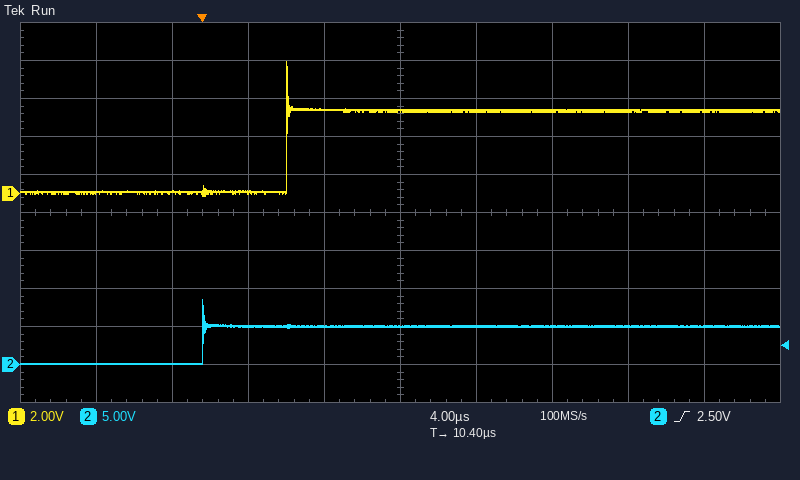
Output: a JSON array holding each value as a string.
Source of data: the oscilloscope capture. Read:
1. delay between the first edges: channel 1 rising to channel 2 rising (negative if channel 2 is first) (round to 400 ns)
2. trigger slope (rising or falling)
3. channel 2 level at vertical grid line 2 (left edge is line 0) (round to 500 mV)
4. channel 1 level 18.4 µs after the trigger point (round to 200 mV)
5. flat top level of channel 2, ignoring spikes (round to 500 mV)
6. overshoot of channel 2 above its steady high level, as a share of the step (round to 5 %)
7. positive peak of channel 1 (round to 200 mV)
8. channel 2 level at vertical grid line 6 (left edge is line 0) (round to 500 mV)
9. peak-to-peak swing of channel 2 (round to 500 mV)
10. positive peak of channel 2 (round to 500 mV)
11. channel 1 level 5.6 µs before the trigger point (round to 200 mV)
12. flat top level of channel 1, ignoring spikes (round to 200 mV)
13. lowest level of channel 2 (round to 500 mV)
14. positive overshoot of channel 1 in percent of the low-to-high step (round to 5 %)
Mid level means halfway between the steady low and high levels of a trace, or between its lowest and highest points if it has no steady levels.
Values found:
["-4.4 µs", "rising", "0.0 V", "4.4 V", "5.0 V", "70 %", "7.0 V", "5.0 V", "8.5 V", "8.5 V", "0.0 V", "4.4 V", "0.0 V", "60 %"]
